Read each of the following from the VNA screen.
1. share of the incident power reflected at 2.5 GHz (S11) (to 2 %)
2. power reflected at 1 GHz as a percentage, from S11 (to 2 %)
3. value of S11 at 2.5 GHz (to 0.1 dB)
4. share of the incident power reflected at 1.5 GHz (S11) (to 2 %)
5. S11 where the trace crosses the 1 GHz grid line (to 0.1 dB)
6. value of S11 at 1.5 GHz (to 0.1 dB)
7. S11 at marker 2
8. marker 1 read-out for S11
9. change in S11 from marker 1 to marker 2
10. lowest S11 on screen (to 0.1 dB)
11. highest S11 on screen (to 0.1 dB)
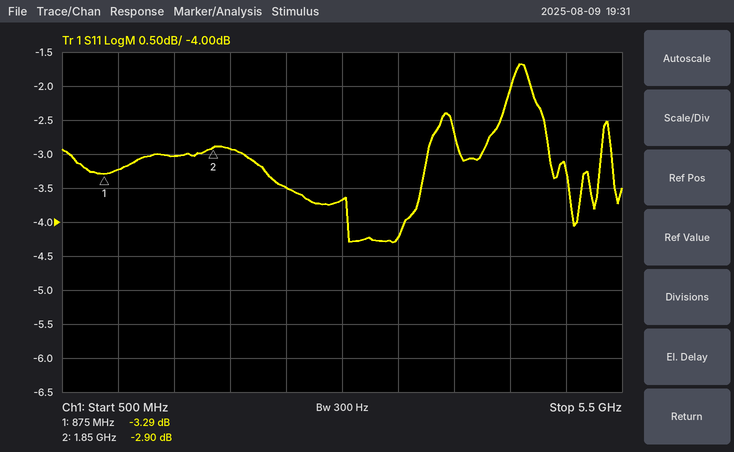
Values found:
44 %
48 %
-3.5 dB
50 %
-3.2 dB
-3.0 dB
-2.90 dB
-3.29 dB
0.39 dB
-4.3 dB
-1.7 dB
